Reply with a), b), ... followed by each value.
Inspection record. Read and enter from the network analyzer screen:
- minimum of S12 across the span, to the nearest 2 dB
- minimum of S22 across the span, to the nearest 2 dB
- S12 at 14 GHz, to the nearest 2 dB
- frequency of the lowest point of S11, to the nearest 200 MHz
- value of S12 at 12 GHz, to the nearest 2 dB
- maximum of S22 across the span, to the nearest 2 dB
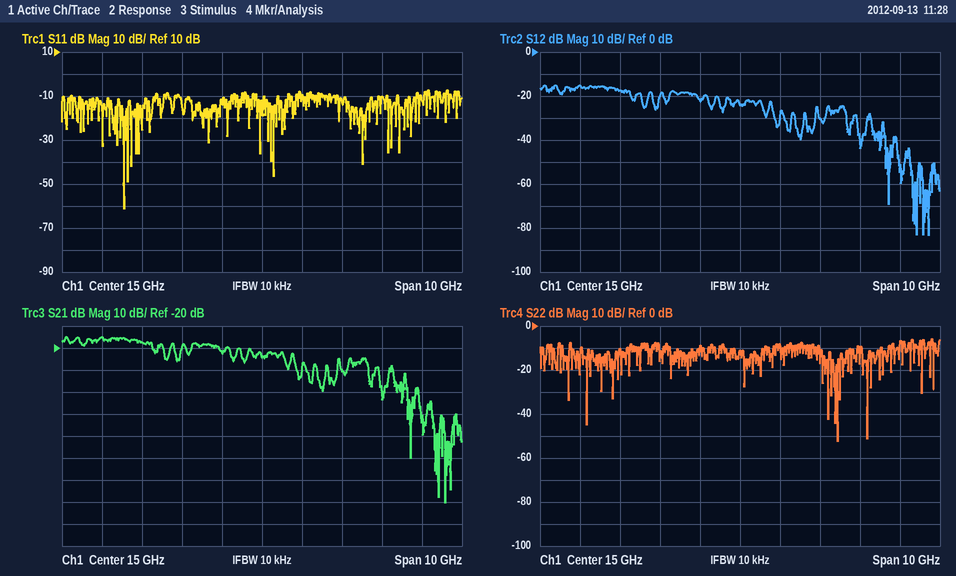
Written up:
a) -84 dB
b) -52 dB
c) -22 dB
d) 11.6 GHz
e) -18 dB
f) -6 dB
